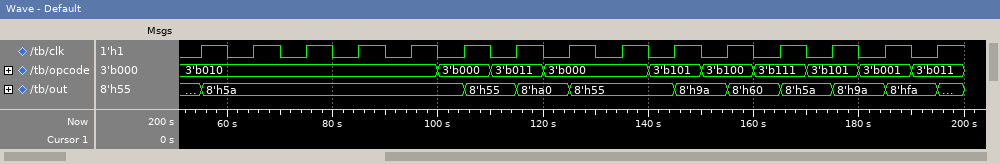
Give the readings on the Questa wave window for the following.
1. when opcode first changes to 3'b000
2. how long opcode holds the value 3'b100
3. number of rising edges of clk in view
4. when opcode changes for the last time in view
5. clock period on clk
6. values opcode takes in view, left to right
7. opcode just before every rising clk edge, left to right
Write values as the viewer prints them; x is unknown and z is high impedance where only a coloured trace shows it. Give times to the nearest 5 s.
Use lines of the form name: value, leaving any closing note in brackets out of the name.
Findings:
when opcode first changes to 3'b000: 100 s
how long opcode holds the value 3'b100: 10 s
number of rising edges of clk in view: 15
when opcode changes for the last time in view: 190 s
clock period on clk: 10 s
values opcode takes in view, left to right: 3'b010, 3'b000, 3'b011, 3'b000, 3'b101, 3'b100, 3'b111, 3'b101, 3'b001, 3'b011
opcode just before every rising clk edge, left to right: 3'b010, 3'b010, 3'b010, 3'b010, 3'b010, 3'b000, 3'b011, 3'b000, 3'b000, 3'b101, 3'b100, 3'b111, 3'b101, 3'b001, 3'b011
